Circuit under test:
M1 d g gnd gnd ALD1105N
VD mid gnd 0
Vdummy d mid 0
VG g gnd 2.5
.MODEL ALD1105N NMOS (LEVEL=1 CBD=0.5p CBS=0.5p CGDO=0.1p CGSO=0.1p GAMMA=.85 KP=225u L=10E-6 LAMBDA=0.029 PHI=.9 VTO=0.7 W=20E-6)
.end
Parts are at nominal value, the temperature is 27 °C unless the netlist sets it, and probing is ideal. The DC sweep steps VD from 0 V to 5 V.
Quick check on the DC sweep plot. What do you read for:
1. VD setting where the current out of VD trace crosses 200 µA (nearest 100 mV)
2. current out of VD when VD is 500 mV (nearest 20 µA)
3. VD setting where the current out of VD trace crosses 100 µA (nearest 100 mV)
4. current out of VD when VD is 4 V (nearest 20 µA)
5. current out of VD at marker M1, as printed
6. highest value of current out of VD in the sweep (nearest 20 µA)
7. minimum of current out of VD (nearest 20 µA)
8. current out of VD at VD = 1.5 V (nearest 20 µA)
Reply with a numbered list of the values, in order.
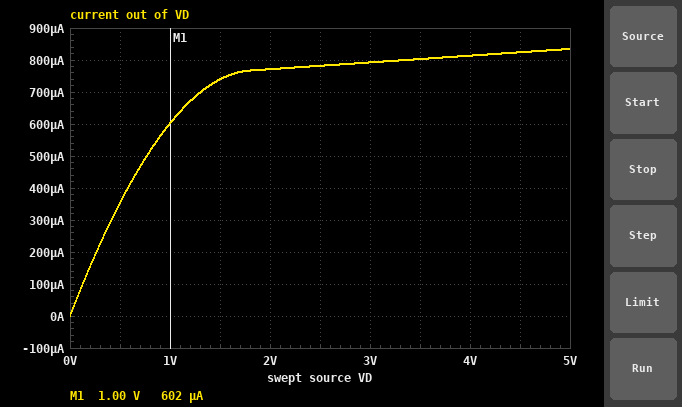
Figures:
1. 300 mV
2. 360 µA
3. 100 mV
4. 820 µA
5. 602 µA
6. 840 µA
7. 0 A
8. 740 µA
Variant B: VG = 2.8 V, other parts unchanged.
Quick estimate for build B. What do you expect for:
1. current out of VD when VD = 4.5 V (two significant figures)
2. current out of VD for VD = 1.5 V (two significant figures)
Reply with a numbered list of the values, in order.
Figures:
1. 1.1 mA
2. 950 µA
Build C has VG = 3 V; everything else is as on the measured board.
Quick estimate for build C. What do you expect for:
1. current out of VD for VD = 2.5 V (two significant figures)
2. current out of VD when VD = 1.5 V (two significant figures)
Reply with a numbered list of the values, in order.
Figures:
1. 1.3 mA
2. 1.1 mA
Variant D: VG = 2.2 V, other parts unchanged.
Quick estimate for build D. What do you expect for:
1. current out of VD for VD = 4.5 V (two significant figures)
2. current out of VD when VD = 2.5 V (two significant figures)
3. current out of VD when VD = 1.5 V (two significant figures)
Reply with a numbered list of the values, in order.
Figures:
1. 570 µA
2. 540 µA
3. 530 µA
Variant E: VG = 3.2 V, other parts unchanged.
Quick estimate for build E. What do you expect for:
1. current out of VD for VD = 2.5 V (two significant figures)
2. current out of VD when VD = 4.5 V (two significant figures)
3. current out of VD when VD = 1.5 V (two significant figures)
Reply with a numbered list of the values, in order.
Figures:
1. 1.5 mA
2. 1.6 mA
3. 1.2 mA
